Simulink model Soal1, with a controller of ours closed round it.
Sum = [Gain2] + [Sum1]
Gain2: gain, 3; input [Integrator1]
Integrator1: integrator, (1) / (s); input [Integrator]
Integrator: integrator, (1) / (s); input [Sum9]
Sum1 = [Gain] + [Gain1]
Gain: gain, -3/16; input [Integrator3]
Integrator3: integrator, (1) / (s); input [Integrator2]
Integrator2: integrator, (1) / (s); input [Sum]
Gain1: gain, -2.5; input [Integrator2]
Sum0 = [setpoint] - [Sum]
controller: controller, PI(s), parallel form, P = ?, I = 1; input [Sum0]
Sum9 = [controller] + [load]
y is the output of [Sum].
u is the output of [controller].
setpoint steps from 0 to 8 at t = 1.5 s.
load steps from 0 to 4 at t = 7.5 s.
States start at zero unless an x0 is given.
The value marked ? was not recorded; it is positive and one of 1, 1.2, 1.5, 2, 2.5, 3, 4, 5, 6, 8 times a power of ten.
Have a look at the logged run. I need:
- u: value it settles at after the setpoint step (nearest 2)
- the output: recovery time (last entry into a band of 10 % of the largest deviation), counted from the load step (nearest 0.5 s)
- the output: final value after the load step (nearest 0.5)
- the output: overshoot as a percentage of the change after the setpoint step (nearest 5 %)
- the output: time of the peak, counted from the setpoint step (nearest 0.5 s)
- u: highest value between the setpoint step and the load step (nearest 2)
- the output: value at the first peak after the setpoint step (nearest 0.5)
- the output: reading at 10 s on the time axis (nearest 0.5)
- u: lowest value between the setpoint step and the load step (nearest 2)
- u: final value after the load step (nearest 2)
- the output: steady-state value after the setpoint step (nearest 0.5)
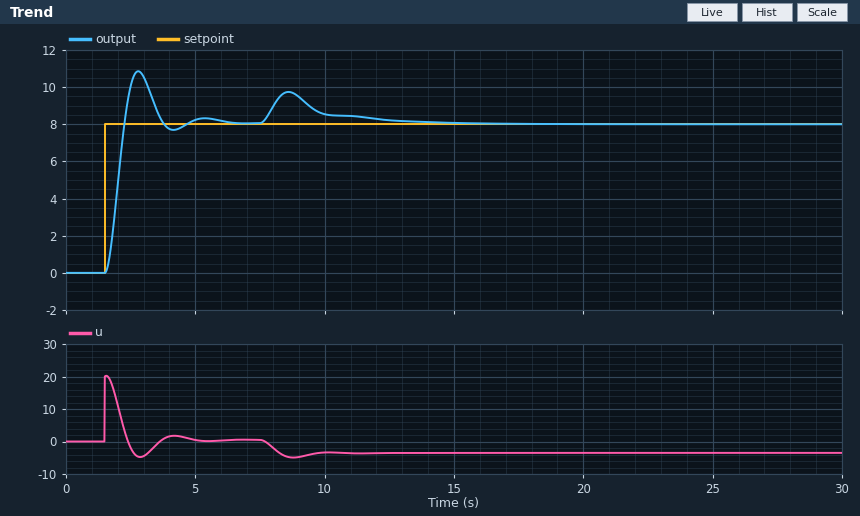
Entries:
0
5.5 s
8.0
35 %
1.5 s
20
11.0
8.5
-4
-4
8.0
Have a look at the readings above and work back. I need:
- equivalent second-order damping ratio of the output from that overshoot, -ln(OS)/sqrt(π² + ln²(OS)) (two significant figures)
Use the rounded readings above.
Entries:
0.32
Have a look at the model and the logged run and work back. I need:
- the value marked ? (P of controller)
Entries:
2.5
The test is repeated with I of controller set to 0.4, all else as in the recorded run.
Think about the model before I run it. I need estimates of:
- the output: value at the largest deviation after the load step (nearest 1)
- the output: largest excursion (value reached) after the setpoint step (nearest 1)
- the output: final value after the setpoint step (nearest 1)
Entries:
10
10
8
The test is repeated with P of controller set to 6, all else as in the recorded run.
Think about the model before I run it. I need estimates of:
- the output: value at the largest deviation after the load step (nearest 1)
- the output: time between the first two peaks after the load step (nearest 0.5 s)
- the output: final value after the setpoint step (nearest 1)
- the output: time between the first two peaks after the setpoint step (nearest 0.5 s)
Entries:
9
1.5 s
8
1.5 s
